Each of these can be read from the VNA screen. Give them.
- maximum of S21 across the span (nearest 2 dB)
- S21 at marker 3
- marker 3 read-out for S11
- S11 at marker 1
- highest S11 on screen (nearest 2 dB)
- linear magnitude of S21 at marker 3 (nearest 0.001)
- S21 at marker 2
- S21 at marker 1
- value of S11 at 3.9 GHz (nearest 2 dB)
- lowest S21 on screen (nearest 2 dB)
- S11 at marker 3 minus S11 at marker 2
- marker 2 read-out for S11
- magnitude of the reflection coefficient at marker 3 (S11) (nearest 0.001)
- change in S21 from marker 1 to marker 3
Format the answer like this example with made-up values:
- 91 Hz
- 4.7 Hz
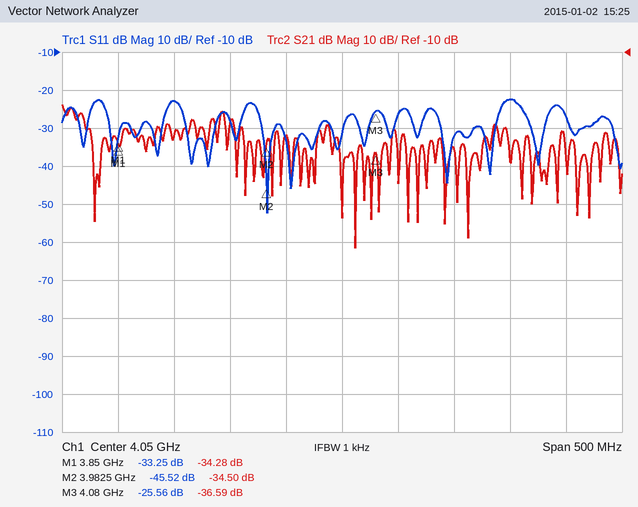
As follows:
- -24 dB
- -36.59 dB
- -25.56 dB
- -33.25 dB
- -22 dB
- 0.015
- -34.50 dB
- -34.28 dB
- -22 dB
- -62 dB
- 19.96 dB
- -45.52 dB
- 0.053
- -2.31 dB
